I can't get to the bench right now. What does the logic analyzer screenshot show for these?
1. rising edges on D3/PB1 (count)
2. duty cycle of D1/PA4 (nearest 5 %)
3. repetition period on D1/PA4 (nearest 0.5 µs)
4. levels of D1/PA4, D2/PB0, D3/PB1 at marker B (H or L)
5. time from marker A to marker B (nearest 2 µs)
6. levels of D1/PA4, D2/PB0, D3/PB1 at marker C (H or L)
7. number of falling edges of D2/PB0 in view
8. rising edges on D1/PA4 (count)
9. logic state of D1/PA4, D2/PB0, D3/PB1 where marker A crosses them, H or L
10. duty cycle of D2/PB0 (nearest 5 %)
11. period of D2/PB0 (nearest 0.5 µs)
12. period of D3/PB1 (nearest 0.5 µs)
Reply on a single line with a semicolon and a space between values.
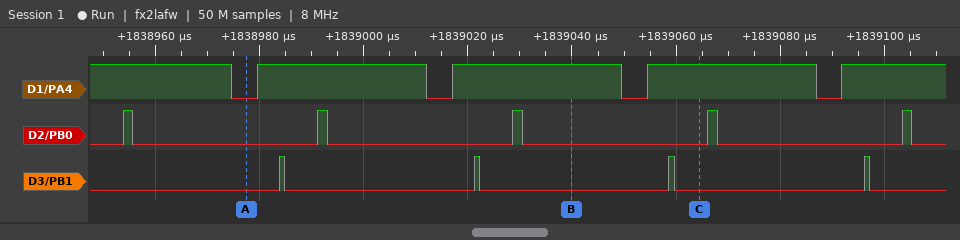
4; 85 %; 37.5 µs; D1/PA4=H, D2/PB0=L, D3/PB1=L; 62 µs; D1/PA4=H, D2/PB0=L, D3/PB1=L; 5; 4; D1/PA4=L, D2/PB0=L, D3/PB1=L; 5 %; 37.5 µs; 37.5 µs
